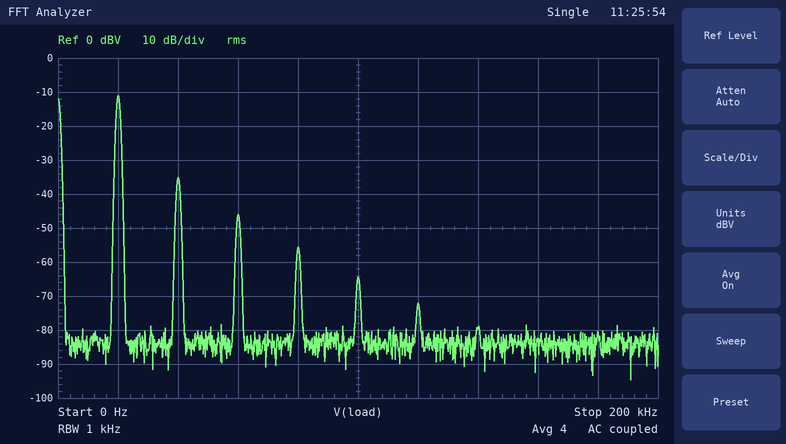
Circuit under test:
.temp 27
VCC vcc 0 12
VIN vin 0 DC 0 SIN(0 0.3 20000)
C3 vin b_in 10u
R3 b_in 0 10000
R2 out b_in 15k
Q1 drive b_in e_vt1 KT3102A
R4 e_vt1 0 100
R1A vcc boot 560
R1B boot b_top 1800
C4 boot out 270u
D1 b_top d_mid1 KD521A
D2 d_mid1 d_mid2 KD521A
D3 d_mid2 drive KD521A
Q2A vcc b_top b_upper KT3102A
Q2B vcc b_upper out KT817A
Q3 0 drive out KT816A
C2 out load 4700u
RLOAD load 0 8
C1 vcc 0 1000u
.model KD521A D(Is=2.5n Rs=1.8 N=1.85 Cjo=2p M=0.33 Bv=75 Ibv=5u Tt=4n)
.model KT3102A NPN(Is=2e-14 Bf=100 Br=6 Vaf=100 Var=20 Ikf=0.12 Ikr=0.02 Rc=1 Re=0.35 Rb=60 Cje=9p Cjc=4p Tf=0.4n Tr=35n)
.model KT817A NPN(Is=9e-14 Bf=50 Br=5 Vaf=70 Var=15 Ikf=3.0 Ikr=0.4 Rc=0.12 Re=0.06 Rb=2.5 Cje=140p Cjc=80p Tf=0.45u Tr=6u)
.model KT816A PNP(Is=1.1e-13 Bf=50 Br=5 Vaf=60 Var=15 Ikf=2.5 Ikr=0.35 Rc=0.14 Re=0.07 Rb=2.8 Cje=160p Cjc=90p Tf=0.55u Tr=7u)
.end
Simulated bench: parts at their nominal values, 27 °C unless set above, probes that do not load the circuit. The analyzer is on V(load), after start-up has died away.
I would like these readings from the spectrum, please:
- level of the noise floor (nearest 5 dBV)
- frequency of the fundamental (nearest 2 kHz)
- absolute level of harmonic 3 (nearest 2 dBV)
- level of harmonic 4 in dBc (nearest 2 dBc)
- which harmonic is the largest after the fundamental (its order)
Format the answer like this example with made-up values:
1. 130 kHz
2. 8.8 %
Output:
1. -85 dBV
2. 20 kHz
3. -46 dBV
4. -44 dBc
5. 2
